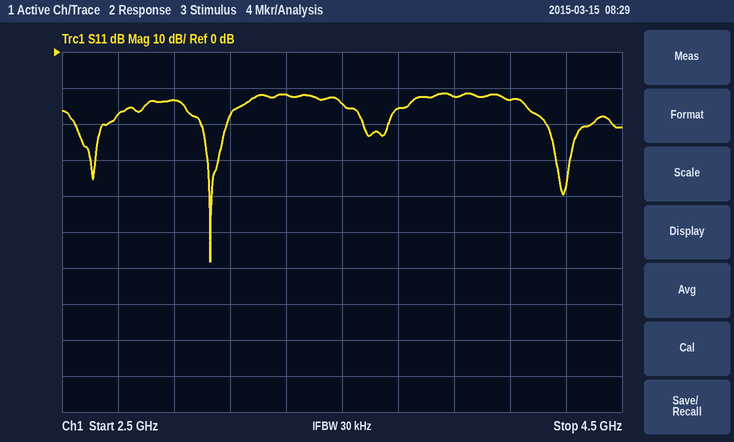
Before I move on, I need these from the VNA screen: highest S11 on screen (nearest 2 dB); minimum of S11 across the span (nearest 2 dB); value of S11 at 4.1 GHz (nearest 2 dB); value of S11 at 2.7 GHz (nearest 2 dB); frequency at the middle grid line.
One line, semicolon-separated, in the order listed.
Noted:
-12 dB; -58 dB; -14 dB; -18 dB; 3.5 GHz
